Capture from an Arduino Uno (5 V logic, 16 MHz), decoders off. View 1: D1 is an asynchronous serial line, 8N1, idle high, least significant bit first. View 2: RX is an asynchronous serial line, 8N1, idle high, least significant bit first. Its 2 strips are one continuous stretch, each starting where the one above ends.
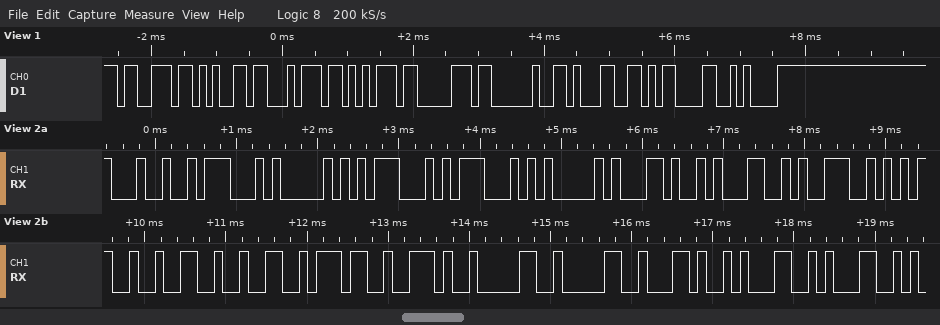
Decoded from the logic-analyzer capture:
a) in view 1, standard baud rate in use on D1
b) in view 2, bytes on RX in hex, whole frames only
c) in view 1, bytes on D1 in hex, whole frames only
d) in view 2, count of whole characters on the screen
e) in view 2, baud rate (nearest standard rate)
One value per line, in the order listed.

9600 baud
24 47 50 47 47 41 2C 31 39 35 32 32 37 2E 30 30 2C 31 31
73 65 74 75 70 20 31 0D 0A
19
9600 baud
